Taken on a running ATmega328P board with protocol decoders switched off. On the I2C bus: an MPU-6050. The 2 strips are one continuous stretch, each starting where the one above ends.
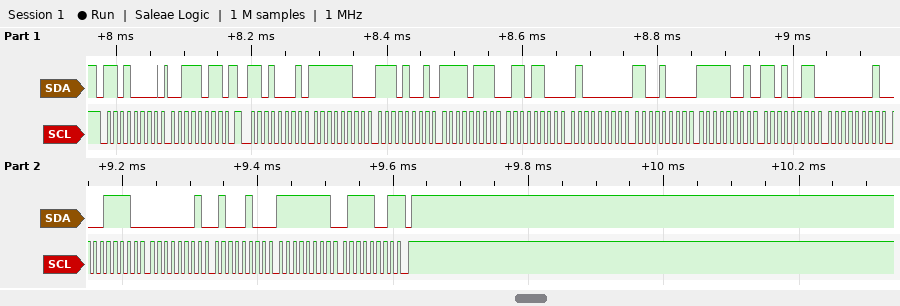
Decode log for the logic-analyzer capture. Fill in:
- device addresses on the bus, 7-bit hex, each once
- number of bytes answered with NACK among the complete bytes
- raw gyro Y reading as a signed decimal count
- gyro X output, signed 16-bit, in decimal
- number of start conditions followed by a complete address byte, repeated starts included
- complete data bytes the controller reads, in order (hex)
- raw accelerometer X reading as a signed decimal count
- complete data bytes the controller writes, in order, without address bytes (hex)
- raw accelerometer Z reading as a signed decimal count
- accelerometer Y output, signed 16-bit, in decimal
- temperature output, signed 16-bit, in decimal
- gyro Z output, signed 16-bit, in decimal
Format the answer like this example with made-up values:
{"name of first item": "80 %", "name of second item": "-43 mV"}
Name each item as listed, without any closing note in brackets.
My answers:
{"device addresses on the bus, 7-bit hex, each once": "0x68", "number of bytes answered with NACK among the complete bytes": "1", "raw gyro Y reading as a signed decimal count": "324", "gyro X output, signed 16-bit, in decimal": "286", "number of start conditions followed by a complete address byte, repeated starts included": "2", "complete data bytes the controller reads, in order": "FC E9 F7 6C 40 C8 F9 D3 01 1E 01 44 FF 79", "raw accelerometer X reading as a signed decimal count": "-791", "complete data bytes the controller writes, in order, without address bytes": "3B", "raw accelerometer Z reading as a signed decimal count": "16584", "accelerometer Y output, signed 16-bit, in decimal": "-2196", "temperature output, signed 16-bit, in decimal": "-1581", "gyro Z output, signed 16-bit, in decimal": "-135"}
